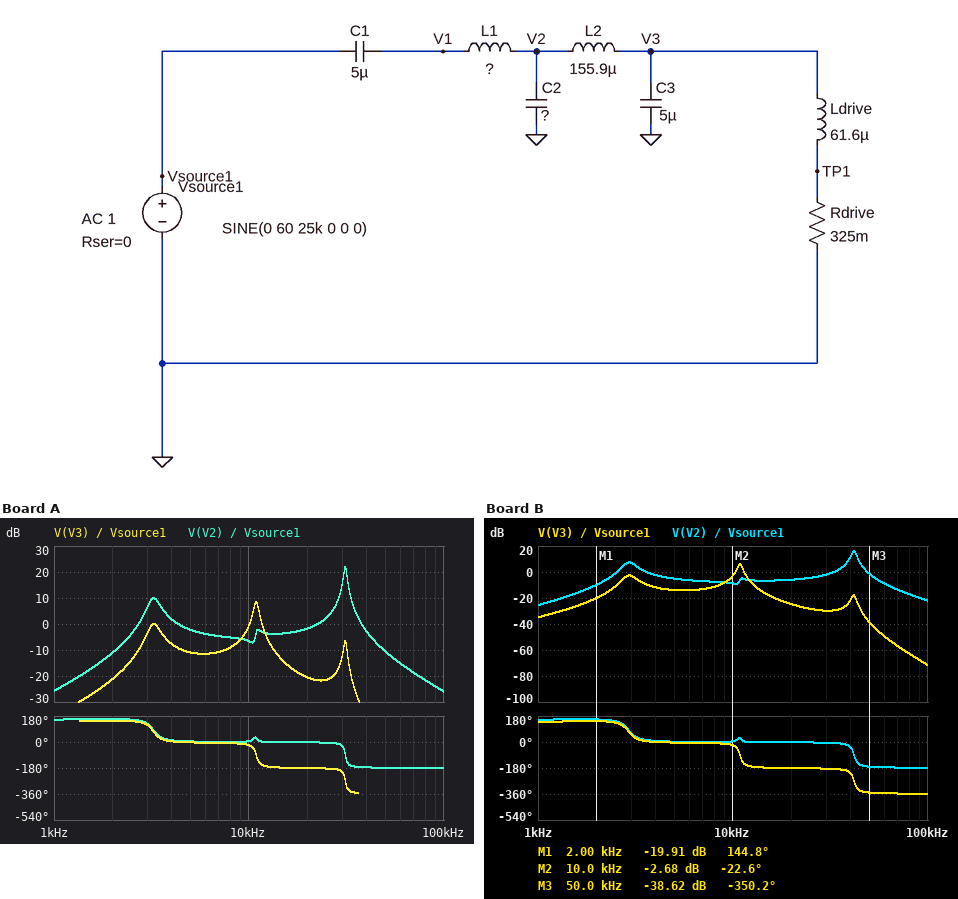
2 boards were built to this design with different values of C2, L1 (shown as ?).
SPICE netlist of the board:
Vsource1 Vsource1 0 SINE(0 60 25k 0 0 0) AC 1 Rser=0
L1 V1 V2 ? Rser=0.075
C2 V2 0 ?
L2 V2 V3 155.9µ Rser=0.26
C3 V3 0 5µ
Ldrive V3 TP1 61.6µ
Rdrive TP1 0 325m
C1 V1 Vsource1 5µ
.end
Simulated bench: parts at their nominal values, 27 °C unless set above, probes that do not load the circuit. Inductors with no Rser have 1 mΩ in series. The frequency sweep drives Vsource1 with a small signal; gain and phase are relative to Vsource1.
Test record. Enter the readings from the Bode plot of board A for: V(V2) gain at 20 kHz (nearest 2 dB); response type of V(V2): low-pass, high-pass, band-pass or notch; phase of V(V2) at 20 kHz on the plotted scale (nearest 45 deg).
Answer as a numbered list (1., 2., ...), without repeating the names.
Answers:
1. -2 dB
2. band-pass
3. 0 deg
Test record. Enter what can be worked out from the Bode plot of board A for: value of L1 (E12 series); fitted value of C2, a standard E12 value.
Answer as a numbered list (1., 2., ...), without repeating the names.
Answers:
1. 10 µH
2. 5.6 µF
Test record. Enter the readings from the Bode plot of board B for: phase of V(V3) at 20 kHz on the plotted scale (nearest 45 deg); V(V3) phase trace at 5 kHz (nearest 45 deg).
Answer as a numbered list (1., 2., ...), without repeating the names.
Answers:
1. -180 deg
2. 0 deg
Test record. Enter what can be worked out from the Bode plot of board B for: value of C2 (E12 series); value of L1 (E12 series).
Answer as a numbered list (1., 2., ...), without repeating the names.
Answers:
1. 8.2 µF
2. 4.7 µH
